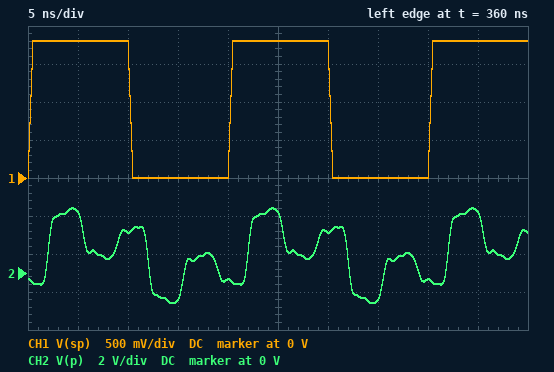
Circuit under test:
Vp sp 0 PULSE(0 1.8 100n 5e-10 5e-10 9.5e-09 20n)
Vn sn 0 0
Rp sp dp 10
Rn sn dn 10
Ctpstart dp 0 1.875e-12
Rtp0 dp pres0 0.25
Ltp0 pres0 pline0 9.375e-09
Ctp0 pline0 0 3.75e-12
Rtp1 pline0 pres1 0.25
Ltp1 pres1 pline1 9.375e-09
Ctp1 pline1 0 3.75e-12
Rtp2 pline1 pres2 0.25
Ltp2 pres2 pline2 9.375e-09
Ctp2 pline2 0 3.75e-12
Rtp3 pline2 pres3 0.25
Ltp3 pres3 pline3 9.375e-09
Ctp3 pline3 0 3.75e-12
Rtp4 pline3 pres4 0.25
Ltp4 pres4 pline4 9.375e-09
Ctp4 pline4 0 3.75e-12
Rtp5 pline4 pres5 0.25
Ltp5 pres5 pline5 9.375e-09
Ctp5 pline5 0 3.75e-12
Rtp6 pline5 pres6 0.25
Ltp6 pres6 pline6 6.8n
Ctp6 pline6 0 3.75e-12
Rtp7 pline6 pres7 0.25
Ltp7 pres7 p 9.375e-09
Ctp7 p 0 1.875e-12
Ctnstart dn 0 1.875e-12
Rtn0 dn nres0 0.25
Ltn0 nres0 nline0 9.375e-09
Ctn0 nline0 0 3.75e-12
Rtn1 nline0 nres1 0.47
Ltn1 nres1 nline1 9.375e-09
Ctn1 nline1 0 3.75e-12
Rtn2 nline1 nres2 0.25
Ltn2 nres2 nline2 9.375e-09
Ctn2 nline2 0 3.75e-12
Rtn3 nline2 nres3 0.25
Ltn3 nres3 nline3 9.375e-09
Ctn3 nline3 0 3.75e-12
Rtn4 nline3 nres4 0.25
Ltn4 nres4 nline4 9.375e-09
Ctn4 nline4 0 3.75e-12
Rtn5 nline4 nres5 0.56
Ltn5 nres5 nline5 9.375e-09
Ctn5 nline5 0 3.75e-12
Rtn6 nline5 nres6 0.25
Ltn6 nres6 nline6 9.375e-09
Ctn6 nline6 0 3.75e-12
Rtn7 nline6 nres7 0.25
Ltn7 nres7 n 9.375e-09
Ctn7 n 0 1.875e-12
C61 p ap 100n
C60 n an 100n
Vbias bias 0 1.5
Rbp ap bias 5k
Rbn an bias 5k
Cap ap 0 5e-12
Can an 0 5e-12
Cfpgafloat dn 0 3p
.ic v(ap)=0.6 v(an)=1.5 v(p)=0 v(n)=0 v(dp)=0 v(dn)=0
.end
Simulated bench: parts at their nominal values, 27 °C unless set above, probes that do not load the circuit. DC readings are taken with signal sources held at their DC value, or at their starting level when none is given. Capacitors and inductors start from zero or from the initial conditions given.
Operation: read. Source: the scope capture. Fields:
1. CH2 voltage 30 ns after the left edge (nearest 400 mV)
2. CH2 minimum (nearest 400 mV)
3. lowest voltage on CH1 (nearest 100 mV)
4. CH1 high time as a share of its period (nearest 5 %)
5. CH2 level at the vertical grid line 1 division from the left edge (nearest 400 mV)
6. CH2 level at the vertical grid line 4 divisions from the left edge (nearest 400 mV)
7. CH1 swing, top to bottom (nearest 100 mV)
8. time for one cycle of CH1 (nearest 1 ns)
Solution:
2.0 V
-1.6 V
0 V
50 %
3.2 V
-400 mV
1.8 V
20 ns
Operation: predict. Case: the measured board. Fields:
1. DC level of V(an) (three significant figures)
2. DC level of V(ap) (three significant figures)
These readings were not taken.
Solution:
1.50 V
1.50 V
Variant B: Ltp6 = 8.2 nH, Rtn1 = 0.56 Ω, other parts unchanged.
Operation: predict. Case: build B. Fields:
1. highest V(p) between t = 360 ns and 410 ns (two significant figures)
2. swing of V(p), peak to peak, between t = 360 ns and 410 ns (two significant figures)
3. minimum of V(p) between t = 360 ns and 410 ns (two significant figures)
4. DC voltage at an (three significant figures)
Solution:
3.3 V
4.9 V
-1.5 V
1.50 V
